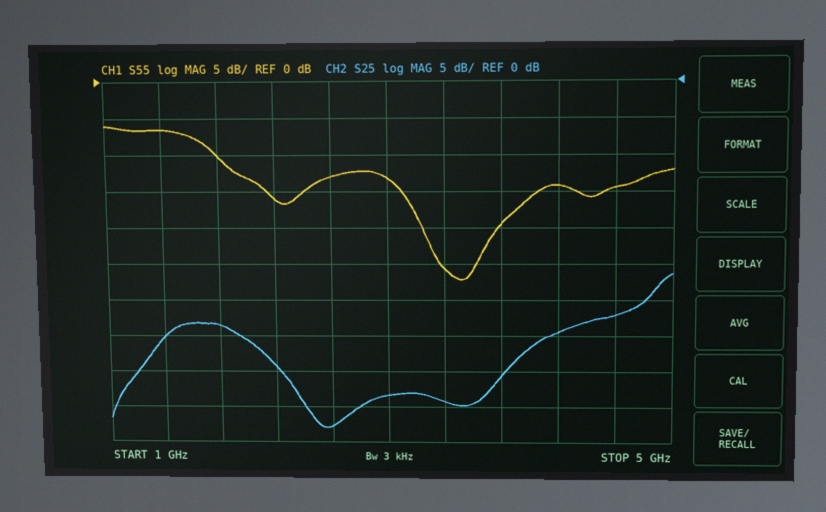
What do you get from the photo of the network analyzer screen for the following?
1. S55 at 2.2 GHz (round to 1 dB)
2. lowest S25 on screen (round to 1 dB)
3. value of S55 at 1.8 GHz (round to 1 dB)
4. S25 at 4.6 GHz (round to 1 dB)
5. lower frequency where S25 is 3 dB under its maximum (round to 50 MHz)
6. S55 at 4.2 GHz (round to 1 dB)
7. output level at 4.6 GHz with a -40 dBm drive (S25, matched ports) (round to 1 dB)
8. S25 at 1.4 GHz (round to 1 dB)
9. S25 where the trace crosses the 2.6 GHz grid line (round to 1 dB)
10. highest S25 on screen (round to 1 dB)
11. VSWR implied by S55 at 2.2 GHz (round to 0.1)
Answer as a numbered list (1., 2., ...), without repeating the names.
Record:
1. -16 dB
2. -48 dB
3. -10 dB
4. -32 dB
5. 4.85 GHz
6. -14 dB
7. -72 dBm
8. -35 dB
9. -48 dB
10. -26 dB
11. 1.4
